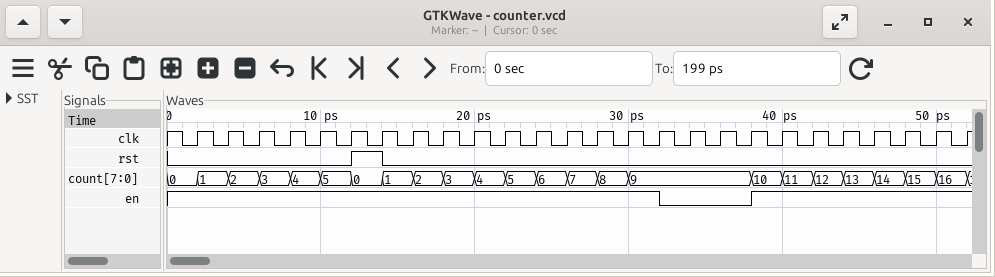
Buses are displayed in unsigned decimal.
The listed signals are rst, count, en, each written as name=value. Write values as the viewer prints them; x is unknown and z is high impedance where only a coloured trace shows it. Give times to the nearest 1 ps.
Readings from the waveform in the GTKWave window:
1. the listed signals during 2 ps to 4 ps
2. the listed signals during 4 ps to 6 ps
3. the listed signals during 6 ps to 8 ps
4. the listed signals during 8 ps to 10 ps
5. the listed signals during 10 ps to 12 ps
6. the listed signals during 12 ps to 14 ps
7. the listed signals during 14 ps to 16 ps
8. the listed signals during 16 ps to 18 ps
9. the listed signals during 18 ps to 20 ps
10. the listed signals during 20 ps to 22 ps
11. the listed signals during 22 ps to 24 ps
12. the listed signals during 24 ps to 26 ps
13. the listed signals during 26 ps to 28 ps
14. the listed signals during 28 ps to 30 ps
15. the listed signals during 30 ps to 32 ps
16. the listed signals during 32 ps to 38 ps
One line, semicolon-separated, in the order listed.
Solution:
rst=0, count=1, en=1; rst=0, count=2, en=1; rst=0, count=3, en=1; rst=0, count=4, en=1; rst=0, count=5, en=1; rst=1, count=0, en=1; rst=0, count=1, en=1; rst=0, count=2, en=1; rst=0, count=3, en=1; rst=0, count=4, en=1; rst=0, count=5, en=1; rst=0, count=6, en=1; rst=0, count=7, en=1; rst=0, count=8, en=1; rst=0, count=9, en=1; rst=0, count=9, en=0
